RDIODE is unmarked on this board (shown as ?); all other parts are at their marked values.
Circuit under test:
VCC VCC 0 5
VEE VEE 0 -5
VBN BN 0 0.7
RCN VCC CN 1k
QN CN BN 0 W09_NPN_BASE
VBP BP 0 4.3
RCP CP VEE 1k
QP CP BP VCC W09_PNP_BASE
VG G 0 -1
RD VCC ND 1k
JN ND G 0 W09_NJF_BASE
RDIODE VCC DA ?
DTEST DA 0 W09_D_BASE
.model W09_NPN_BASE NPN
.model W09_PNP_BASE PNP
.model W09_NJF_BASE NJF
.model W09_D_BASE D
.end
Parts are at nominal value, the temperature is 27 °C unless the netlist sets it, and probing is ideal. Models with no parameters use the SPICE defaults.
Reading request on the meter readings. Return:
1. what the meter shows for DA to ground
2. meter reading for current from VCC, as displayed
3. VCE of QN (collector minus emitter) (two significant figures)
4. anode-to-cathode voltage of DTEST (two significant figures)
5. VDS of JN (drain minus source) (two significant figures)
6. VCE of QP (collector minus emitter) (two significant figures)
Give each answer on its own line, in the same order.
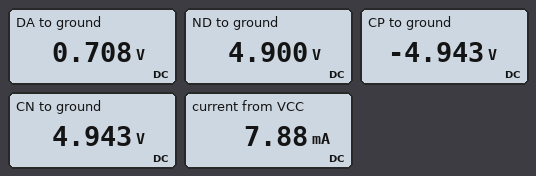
0.708 V
7.88 mA
4.9 V
710 mV
4.9 V
-9.9 V
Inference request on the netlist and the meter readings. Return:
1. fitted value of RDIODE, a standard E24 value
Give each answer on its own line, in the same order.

560 Ω
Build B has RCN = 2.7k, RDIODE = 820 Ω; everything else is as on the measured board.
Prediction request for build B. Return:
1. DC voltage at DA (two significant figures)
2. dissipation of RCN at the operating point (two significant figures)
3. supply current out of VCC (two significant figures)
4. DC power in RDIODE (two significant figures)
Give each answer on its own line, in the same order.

700 mV
8.7 µW
5.5 mA
23 mW
